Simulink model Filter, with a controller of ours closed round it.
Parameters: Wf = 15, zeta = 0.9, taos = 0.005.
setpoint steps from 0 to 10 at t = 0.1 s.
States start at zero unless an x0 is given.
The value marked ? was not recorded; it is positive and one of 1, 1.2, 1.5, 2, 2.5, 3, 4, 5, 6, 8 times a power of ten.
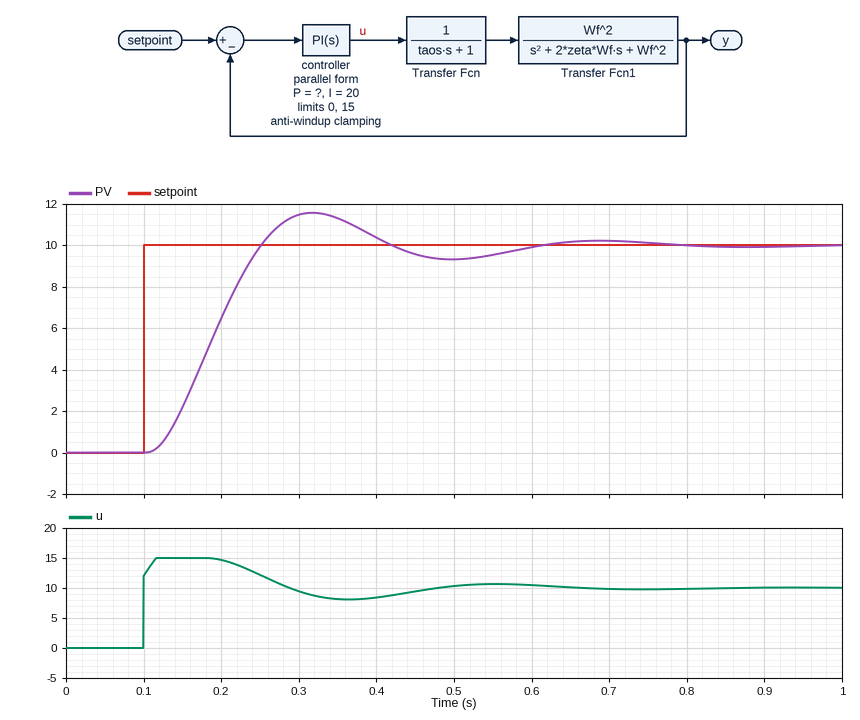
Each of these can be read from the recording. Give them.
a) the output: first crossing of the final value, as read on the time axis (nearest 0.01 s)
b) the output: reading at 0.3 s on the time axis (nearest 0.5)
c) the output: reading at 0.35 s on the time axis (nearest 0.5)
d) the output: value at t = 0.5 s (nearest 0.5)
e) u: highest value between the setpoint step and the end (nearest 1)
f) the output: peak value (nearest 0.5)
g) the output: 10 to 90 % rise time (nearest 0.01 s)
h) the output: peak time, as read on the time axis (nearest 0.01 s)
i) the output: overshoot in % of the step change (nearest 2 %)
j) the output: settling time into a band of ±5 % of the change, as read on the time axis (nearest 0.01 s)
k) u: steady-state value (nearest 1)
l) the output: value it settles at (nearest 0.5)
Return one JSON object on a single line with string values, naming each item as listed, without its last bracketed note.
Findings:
{"the output: first crossing of the final value, as read on the time axis": "0.25 s", "the output: reading at 0.3 s on the time axis": "11.5", "the output: reading at 0.35 s on the time axis": "11.5", "the output: value at t = 0.5 s": "9.5", "u: highest value between the setpoint step and the end": "15", "the output: peak value": "11.5", "the output: 10 to 90 % rise time": "0.10 s", "the output: peak time, as read on the time axis": "0.32 s", "the output: overshoot in % of the step change": "16 %", "the output: settling time into a band of ±5 % of the change, as read on the time axis": "0.54 s", "u: steady-state value": "10", "the output: value it settles at": "10.0"}
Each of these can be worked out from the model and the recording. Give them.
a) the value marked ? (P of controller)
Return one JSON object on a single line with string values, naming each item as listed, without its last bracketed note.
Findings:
{"the value marked ?": "1.2"}
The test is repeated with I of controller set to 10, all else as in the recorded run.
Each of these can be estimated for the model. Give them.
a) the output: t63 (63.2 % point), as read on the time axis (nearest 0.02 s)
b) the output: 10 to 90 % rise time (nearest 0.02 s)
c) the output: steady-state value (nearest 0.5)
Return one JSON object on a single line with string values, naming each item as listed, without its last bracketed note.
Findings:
{"the output: t63 (63.2 % point), as read on the time axis": "0.20 s", "the output: 10 to 90 % rise time": "0.12 s", "the output: steady-state value": "10.0"}
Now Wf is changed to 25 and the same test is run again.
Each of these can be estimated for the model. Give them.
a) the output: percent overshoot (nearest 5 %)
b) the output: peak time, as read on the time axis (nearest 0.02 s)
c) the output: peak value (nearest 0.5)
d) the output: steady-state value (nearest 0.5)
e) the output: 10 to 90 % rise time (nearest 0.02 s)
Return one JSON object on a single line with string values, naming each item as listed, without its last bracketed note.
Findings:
{"the output: percent overshoot": "10 %", "the output: peak time, as read on the time axis": "0.24 s", "the output: peak value": "11.0", "the output: steady-state value": "10.0", "the output: 10 to 90 % rise time": "0.06 s"}
